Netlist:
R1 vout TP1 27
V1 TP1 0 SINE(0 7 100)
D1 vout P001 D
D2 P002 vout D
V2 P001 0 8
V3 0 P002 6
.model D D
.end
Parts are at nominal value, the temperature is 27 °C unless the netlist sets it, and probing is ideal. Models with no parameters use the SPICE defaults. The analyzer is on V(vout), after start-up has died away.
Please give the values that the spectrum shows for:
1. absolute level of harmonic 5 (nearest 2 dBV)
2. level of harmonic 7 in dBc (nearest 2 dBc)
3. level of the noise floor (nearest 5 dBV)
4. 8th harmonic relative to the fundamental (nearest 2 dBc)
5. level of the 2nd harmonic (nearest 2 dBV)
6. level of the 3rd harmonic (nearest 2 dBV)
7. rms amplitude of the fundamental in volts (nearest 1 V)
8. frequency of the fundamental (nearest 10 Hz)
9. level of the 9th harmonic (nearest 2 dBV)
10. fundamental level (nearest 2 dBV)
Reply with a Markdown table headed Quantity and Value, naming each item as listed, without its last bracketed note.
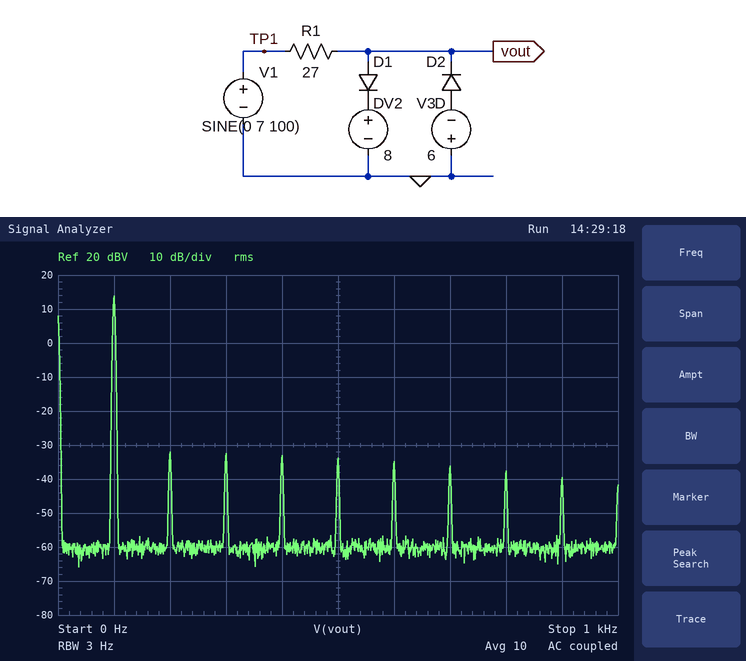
| Quantity | Value |
|---|---|
| absolute level of harmonic 5 | -34 dBV |
| level of harmonic 7 in dBc | -50 dBc |
| level of the noise floor | -60 dBV |
| 8th harmonic relative to the fundamental | -52 dBc |
| level of the 2nd harmonic | -32 dBV |
| level of the 3rd harmonic | -32 dBV |
| rms amplitude of the fundamental in volts | 5 V |
| frequency of the fundamental | 100 Hz |
| level of the 9th harmonic | -40 dBV |
| fundamental level | 14 dBV |
